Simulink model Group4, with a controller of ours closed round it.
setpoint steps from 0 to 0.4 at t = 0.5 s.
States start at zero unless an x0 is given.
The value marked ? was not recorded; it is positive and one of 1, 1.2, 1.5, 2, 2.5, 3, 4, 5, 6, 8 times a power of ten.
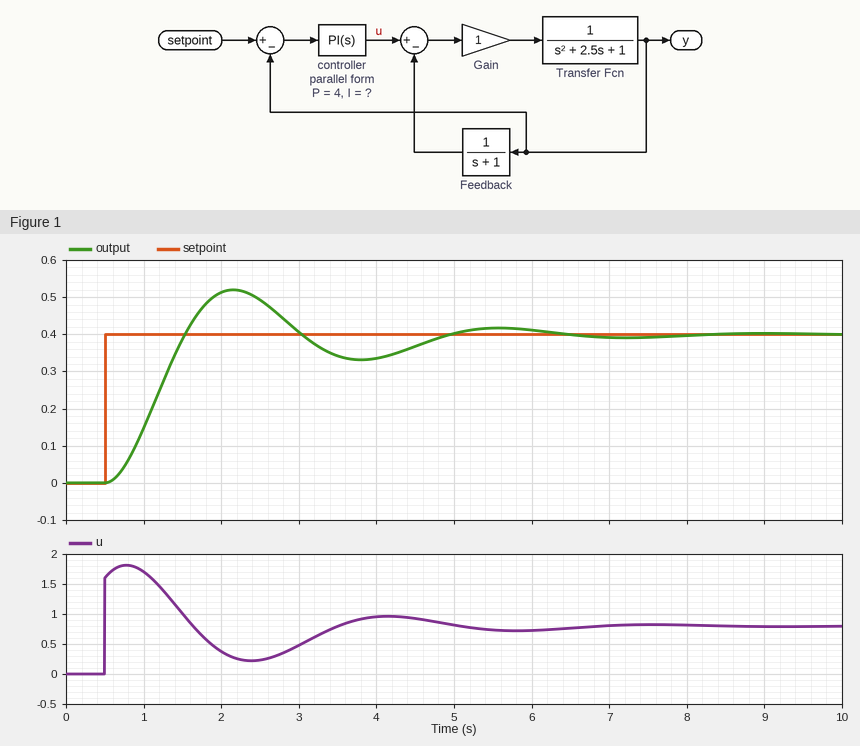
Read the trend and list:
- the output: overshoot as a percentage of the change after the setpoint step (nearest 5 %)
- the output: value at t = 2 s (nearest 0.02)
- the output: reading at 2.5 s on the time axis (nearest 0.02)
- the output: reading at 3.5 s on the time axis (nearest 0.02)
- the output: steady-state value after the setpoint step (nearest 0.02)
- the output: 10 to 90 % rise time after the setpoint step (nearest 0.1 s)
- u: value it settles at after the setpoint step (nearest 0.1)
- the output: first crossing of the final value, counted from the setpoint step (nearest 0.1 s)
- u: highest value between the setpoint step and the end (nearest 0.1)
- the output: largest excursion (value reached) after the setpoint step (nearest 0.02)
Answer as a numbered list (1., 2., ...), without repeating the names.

1. 30 %
2. 0.52
3. 0.50
4. 0.34
5. 0.40
6. 0.7 s
7. 0.8
8. 1.0 s
9. 1.8
10. 0.52
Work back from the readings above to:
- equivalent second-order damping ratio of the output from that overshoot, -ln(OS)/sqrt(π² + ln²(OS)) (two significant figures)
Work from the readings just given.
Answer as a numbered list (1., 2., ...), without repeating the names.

1. 0.36
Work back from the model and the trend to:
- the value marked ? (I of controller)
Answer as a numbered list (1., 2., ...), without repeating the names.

1. 4
